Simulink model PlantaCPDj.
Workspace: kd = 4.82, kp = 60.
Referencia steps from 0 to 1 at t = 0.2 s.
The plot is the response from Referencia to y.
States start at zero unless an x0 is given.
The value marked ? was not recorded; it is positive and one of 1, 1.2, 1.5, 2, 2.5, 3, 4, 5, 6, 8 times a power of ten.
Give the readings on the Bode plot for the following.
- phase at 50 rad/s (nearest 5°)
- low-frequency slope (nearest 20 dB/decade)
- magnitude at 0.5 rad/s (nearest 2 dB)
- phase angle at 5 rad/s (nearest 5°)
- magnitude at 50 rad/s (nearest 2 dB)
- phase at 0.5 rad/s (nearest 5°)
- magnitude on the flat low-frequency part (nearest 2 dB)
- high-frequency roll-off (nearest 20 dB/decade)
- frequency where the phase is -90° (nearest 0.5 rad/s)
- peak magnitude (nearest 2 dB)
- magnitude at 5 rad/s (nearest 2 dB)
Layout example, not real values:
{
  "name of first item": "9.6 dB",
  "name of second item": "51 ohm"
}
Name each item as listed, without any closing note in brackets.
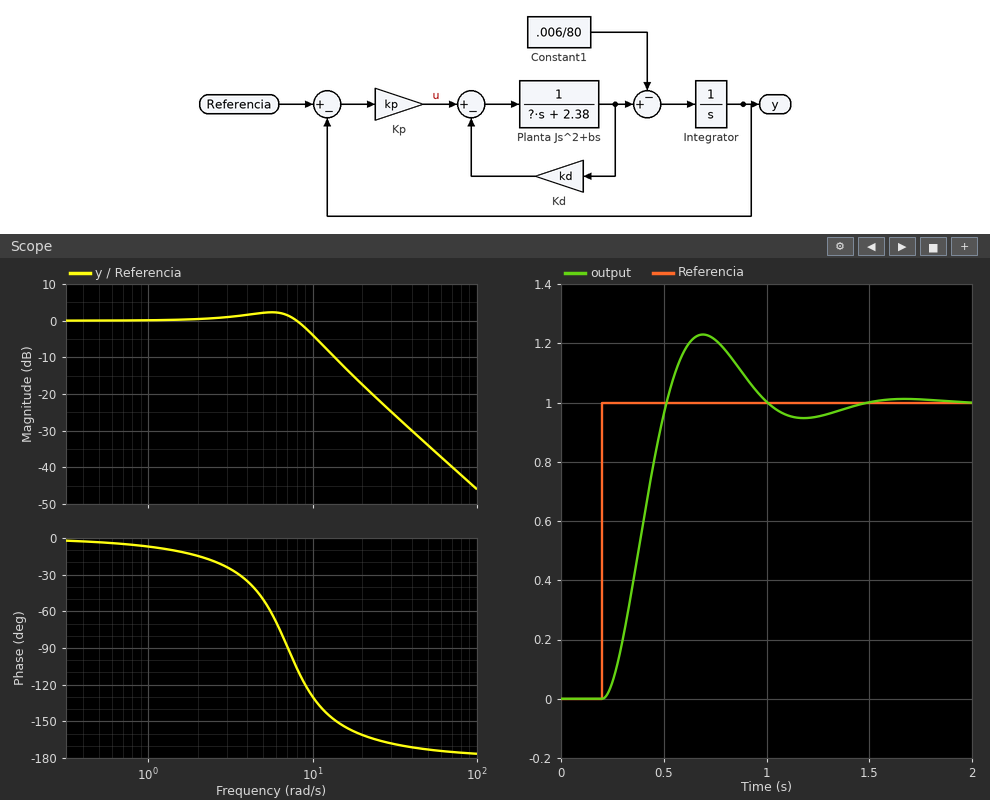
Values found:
{
  "phase at 50 rad/s": "-175°",
  "low-frequency slope": "0 dB/decade",
  "magnitude at 0.5 rad/s": "0 dB",
  "phase angle at 5 rad/s": "-50°",
  "magnitude at 50 rad/s": "-34 dB",
  "phase at 0.5 rad/s": "-5°",
  "magnitude on the flat low-frequency part": "0 dB",
  "high-frequency roll-off": "-40 dB/decade",
  "frequency where the phase is -90°": "7.0 rad/s",
  "peak magnitude": "2 dB",
  "magnitude at 5 rad/s": "2 dB"
}
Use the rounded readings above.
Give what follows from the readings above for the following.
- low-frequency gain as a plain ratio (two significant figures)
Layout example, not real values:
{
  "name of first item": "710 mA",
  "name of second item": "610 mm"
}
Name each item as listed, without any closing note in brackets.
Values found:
{
  "low-frequency gain as a plain ratio": "1.0"
}
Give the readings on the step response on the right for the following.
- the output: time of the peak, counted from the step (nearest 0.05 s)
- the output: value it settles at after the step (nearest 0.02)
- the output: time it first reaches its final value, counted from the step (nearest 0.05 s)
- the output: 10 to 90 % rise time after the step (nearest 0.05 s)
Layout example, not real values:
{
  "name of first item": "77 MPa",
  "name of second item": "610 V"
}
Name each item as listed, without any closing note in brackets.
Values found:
{
  "the output: time of the peak, counted from the step": "0.50 s",
  "the output: value it settles at after the step": "1.00",
  "the output: time it first reaches its final value, counted from the step": "0.30 s",
  "the output: 10 to 90 % rise time after the step": "0.20 s"
}
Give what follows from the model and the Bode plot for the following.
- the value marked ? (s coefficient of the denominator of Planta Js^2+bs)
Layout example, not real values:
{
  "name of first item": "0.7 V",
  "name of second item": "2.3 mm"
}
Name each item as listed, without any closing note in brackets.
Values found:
{
  "the value marked ?": "1.2"
}
